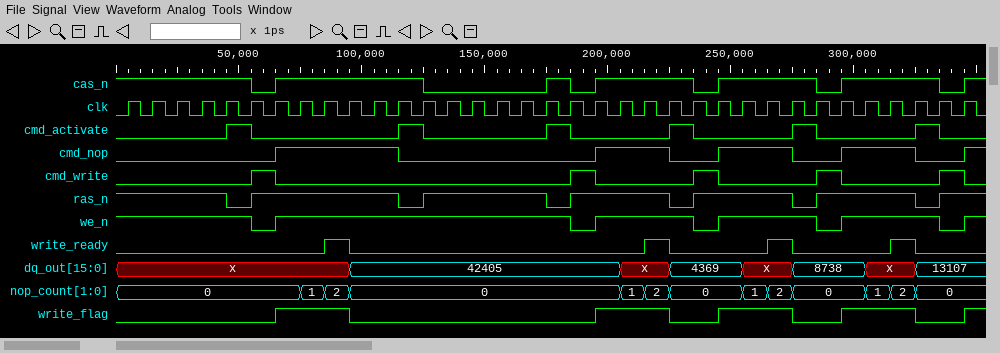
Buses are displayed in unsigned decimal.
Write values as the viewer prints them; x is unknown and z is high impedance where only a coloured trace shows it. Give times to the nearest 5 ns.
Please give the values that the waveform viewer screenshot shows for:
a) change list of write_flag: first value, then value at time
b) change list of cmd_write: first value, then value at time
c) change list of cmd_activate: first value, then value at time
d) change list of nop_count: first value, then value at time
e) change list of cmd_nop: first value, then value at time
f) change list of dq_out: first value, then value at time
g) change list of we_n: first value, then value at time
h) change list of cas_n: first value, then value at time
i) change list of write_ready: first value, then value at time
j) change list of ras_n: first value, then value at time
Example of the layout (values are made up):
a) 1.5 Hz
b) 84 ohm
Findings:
a) 0, 1 at 65 ns, 0 at 95 ns, 1 at 195 ns, 0 at 225 ns, 1 at 245 ns, 0 at 275 ns, 1 at 295 ns, 0 at 325 ns, 1 at 345 ns
b) 0, 1 at 55 ns, 0 at 65 ns, 1 at 185 ns, 0 at 195 ns, 1 at 235 ns, 0 at 245 ns, 1 at 285 ns, 0 at 295 ns, 1 at 335 ns, 0 at 345 ns
c) 0, 1 at 45 ns, 0 at 55 ns, 1 at 115 ns, 0 at 125 ns, 1 at 175 ns, 0 at 185 ns, 1 at 225 ns, 0 at 235 ns, 1 at 275 ns, 0 at 285 ns, 1 at 325 ns, 0 at 335 ns
d) 0, 1 at 75 ns, 2 at 85 ns, 0 at 95 ns, 1 at 205 ns, 2 at 215 ns, 0 at 225 ns, 1 at 255 ns, 2 at 265 ns, 0 at 275 ns, 1 at 305 ns, 2 at 315 ns, 0 at 325 ns
e) 0, 1 at 65 ns, 0 at 115 ns, 1 at 195 ns, 0 at 225 ns, 1 at 245 ns, 0 at 275 ns, 1 at 295 ns, 0 at 325 ns, 1 at 345 ns
f) x, 42405 at 95 ns, x at 205 ns, 4369 at 225 ns, x at 255 ns, 8738 at 275 ns, x at 305 ns, 13107 at 325 ns
g) 1, 0 at 55 ns, 1 at 65 ns, 0 at 185 ns, 1 at 195 ns, 0 at 235 ns, 1 at 245 ns, 0 at 285 ns, 1 at 295 ns, 0 at 335 ns, 1 at 345 ns
h) 1, 0 at 55 ns, 1 at 65 ns, 0 at 125 ns, 1 at 175 ns, 0 at 185 ns, 1 at 195 ns, 0 at 235 ns, 1 at 245 ns, 0 at 285 ns, 1 at 295 ns, 0 at 335 ns, 1 at 345 ns
i) 0, 1 at 85 ns, 0 at 95 ns, 1 at 215 ns, 0 at 225 ns, 1 at 265 ns, 0 at 275 ns, 1 at 315 ns, 0 at 325 ns
j) 1, 0 at 45 ns, 1 at 55 ns, 0 at 115 ns, 1 at 125 ns, 0 at 175 ns, 1 at 185 ns, 0 at 225 ns, 1 at 235 ns, 0 at 275 ns, 1 at 285 ns, 0 at 325 ns, 1 at 335 ns
